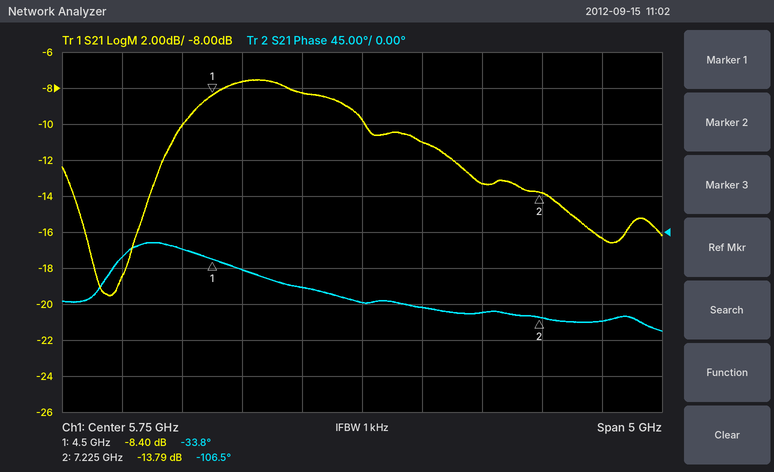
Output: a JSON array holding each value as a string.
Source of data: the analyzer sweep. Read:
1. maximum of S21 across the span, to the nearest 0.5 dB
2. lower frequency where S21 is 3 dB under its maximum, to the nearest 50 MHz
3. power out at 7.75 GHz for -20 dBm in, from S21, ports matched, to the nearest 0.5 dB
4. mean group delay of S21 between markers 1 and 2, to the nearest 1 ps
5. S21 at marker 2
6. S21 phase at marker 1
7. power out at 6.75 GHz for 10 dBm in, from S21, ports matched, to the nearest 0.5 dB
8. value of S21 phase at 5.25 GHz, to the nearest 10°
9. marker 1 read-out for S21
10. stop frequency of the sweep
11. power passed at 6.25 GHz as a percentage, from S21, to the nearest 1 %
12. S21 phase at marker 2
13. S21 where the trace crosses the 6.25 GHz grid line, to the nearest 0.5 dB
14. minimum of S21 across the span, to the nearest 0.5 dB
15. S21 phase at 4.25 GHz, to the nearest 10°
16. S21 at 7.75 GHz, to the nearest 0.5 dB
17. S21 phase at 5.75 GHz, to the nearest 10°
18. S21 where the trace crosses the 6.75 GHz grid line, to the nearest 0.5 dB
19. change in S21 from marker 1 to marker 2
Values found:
["-7.5 dB", "4.20 GHz", "-36.5 dBm", "74 ps", "-13.79 dB", "-33.8°", "-3.5 dBm", "-70°", "-8.40 dB", "8.25 GHz", "8 %", "-106.5°", "-11.0 dB", "-19.5 dB", "-20°", "-16.5 dB", "-90°", "-13.5 dB", "-5.39 dB"]
